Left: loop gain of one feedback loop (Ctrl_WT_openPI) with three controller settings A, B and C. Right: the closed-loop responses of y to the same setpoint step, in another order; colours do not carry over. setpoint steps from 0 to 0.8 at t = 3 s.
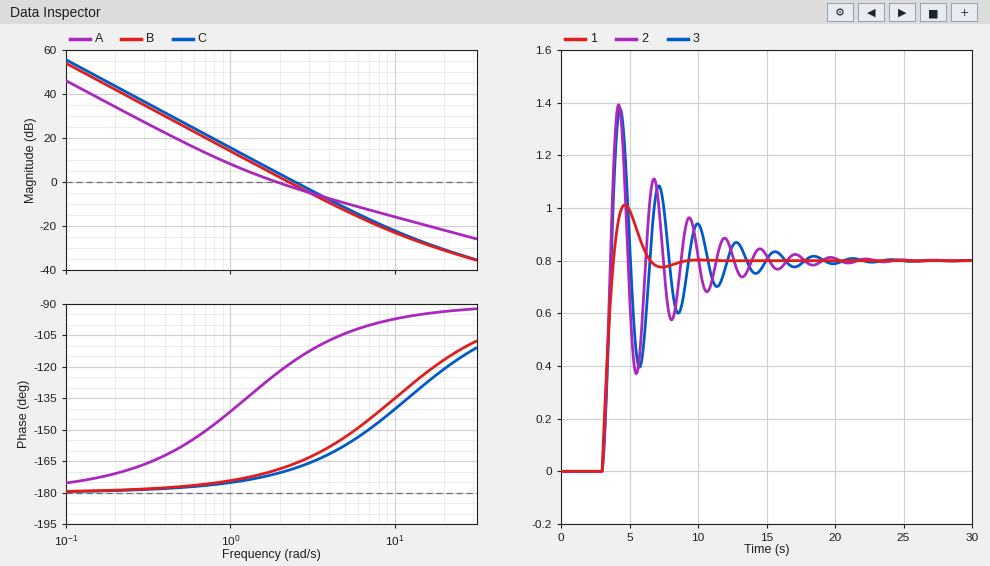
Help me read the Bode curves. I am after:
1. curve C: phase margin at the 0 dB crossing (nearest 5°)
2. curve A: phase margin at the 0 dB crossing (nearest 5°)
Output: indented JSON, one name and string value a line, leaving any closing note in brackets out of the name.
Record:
{
  "curve C: phase margin at the 0 dB crossing": "10°",
  "curve A: phase margin at the 0 dB crossing": "55°"
}
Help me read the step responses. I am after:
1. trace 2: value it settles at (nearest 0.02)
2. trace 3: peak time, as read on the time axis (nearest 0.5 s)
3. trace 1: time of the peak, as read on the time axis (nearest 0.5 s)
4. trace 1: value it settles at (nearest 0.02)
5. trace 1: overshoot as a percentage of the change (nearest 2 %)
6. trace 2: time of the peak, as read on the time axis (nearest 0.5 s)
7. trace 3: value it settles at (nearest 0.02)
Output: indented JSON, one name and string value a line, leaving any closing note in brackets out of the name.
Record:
{
  "trace 2: value it settles at": "0.80",
  "trace 3: peak time, as read on the time axis": "4.5 s",
  "trace 1: time of the peak, as read on the time axis": "4.5 s",
  "trace 1: value it settles at": "0.80",
  "trace 1: overshoot as a percentage of the change": "26 %",
  "trace 2: time of the peak, as read on the time axis": "4.0 s",
  "trace 3: value it settles at": "0.80"
}
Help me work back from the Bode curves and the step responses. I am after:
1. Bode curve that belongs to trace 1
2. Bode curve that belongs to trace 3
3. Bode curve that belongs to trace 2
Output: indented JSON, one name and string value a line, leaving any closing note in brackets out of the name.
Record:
{
  "Bode curve that belongs to trace 1": "A",
  "Bode curve that belongs to trace 3": "B",
  "Bode curve that belongs to trace 2": "C"
}
